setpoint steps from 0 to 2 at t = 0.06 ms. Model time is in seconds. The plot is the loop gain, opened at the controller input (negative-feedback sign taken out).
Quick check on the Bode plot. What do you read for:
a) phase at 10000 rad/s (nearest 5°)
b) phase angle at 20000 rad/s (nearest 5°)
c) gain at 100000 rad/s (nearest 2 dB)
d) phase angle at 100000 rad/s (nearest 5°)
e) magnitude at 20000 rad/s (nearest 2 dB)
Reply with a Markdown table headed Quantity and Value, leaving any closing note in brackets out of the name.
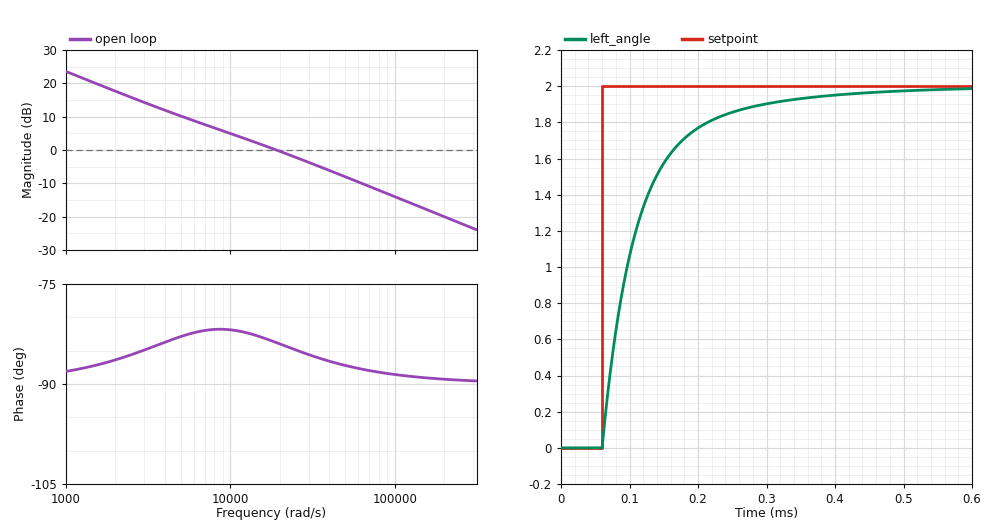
| Quantity | Value |
|---|---|
| phase at 10000 rad/s | -80° |
| phase angle at 20000 rad/s | -85° |
| gain at 100000 rad/s | -14 dB |
| phase angle at 100000 rad/s | -90° |
| magnitude at 20000 rad/s | 0 dB |
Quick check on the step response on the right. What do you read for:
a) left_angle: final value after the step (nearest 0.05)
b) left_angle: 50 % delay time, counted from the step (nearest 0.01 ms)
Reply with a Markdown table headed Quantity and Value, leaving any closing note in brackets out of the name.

| Quantity | Value |
|---|---|
| left_angle: final value after the step | 2.00 |
| left_angle: 50 % delay time, counted from the step | 0.04 ms |
